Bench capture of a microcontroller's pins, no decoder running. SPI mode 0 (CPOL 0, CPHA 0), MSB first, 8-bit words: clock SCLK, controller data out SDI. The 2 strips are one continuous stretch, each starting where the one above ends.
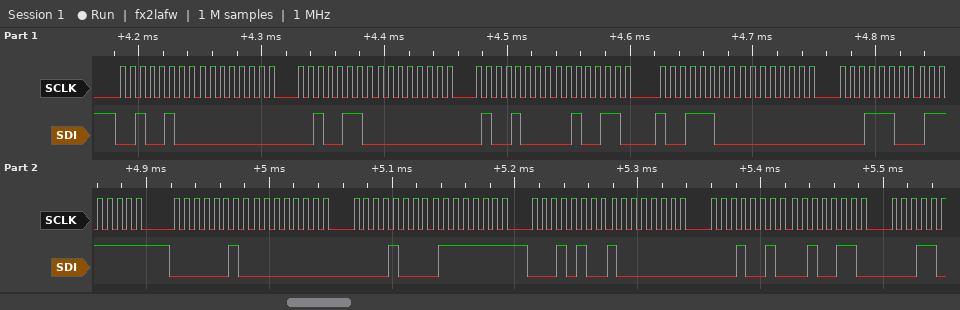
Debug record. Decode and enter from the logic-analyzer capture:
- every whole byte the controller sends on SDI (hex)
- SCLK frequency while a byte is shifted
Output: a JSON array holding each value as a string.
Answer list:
["0x24 0x00 0x26 0x00 0x48 0x26 0x9C 0x00 0x1C 0x7F 0x02 0x00 0x08 0x7F 0x14 0x80 0x12 0x26", "125 kHz"]
